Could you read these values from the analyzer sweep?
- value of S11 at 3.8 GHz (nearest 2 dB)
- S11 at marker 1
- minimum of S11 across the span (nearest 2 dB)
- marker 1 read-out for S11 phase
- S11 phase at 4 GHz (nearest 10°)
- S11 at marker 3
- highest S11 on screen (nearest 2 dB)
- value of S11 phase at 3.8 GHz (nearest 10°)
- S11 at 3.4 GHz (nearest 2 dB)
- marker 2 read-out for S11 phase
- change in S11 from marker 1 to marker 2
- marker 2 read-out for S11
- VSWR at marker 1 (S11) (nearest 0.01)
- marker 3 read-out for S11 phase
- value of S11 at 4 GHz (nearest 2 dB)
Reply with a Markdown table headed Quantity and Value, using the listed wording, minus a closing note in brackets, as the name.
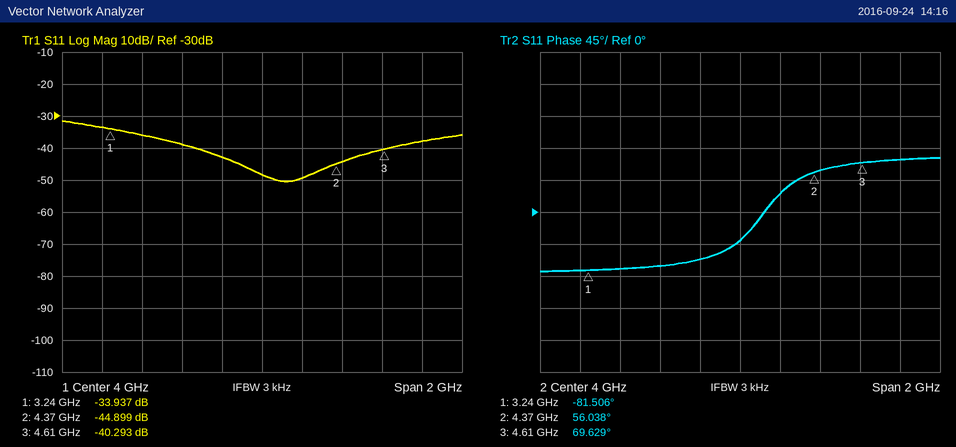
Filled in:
| Quantity | Value |
|---|---|
| value of S11 at 3.8 GHz | -42 dB |
| S11 at marker 1 | -33.937 dB |
| minimum of S11 across the span | -50 dB |
| marker 1 read-out for S11 phase | -81.506° |
| S11 phase at 4 GHz | -40° |
| S11 at marker 3 | -40.293 dB |
| highest S11 on screen | -32 dB |
| value of S11 phase at 3.8 GHz | -70° |
| S11 at 3.4 GHz | -36 dB |
| marker 2 read-out for S11 phase | 56.038° |
| change in S11 from marker 1 to marker 2 | -10.962 dB |
| marker 2 read-out for S11 | -44.899 dB |
| VSWR at marker 1 (S11) | 1.04 |
| marker 3 read-out for S11 phase | 69.629° |
| value of S11 at 4 GHz | -48 dB |
